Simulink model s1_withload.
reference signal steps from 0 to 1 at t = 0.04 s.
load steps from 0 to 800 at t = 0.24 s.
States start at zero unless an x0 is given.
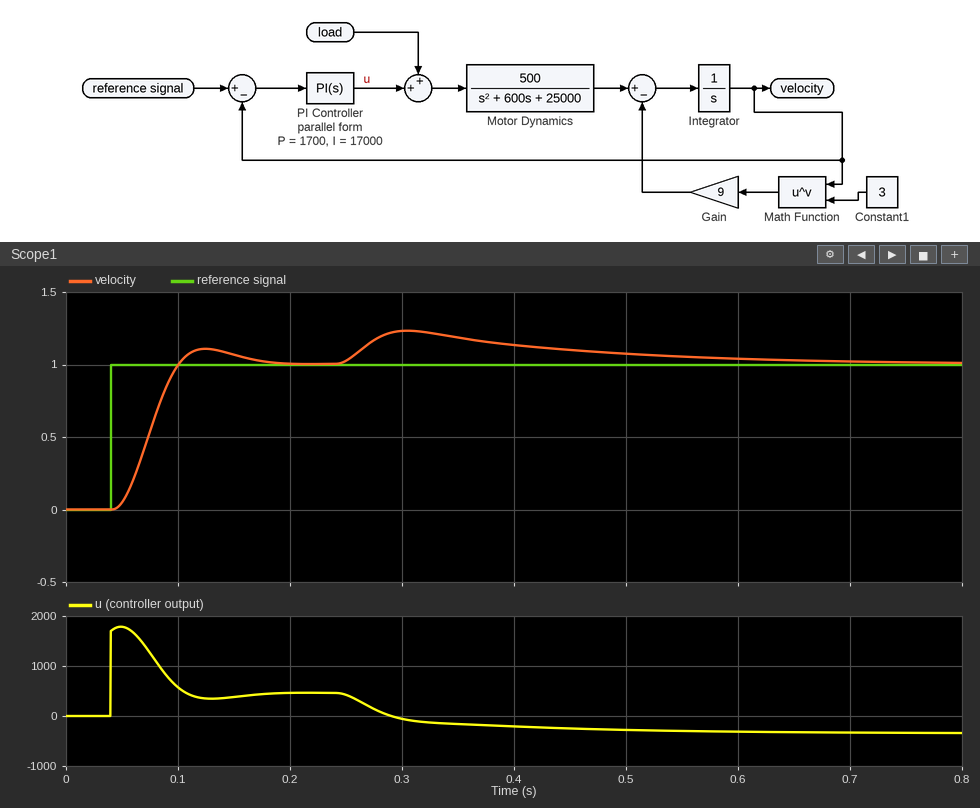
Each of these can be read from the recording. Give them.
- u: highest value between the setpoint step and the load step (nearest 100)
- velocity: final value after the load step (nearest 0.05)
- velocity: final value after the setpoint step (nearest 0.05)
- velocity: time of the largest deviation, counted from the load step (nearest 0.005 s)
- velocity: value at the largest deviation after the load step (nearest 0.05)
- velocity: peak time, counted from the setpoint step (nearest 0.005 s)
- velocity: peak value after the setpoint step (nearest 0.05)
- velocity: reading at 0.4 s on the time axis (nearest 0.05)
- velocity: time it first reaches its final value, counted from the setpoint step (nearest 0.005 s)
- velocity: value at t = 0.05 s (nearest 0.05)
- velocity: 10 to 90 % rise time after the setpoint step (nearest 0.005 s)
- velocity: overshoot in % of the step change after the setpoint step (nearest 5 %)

1800
1.00
1.00
0.065 s
1.25
0.085 s
1.10
1.15
0.060 s
0.05
0.040 s
10 %
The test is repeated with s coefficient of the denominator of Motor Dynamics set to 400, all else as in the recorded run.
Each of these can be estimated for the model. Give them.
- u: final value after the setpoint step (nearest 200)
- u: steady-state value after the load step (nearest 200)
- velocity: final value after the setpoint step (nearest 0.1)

400
-400
1.0
